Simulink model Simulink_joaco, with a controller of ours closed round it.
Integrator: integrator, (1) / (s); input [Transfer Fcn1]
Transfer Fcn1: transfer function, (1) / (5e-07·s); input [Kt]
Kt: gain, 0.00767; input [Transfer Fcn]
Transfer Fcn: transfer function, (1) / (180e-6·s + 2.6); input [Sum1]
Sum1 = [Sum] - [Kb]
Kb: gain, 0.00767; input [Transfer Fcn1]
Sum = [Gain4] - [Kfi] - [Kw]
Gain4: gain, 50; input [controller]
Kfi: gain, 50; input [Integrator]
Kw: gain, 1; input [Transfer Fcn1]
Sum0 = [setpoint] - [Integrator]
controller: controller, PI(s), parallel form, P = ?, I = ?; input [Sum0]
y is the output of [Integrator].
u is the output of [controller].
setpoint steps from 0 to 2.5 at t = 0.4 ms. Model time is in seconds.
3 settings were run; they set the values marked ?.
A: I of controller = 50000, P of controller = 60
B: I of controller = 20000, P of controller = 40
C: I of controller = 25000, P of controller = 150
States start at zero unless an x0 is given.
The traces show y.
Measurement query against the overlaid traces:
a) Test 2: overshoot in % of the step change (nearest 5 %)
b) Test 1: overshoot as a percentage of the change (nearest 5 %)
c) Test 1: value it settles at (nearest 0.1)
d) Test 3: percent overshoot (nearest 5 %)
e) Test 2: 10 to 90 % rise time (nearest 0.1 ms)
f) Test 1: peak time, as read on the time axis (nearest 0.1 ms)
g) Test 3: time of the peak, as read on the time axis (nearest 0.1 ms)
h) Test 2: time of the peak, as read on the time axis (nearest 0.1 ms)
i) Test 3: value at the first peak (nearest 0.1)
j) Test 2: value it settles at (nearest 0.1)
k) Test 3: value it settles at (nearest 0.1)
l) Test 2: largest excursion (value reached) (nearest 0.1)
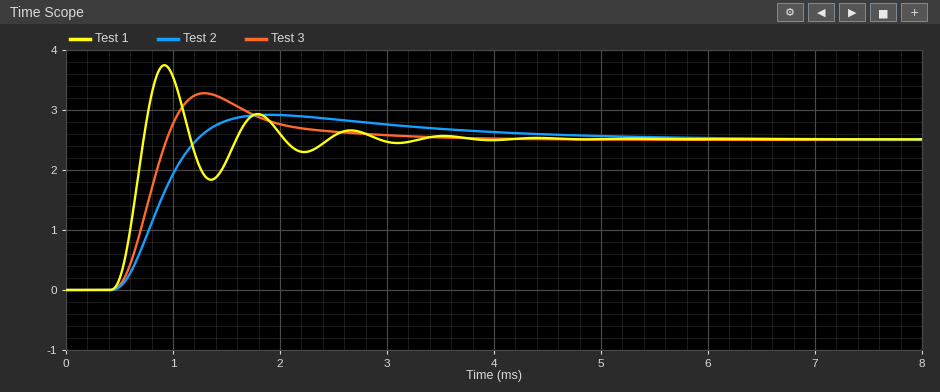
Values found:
15 %
50 %
2.5
30 %
0.5 ms
0.9 ms
1.3 ms
1.9 ms
3.3
2.5
2.5
2.9
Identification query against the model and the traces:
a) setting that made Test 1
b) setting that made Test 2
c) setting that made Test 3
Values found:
C
B
A
